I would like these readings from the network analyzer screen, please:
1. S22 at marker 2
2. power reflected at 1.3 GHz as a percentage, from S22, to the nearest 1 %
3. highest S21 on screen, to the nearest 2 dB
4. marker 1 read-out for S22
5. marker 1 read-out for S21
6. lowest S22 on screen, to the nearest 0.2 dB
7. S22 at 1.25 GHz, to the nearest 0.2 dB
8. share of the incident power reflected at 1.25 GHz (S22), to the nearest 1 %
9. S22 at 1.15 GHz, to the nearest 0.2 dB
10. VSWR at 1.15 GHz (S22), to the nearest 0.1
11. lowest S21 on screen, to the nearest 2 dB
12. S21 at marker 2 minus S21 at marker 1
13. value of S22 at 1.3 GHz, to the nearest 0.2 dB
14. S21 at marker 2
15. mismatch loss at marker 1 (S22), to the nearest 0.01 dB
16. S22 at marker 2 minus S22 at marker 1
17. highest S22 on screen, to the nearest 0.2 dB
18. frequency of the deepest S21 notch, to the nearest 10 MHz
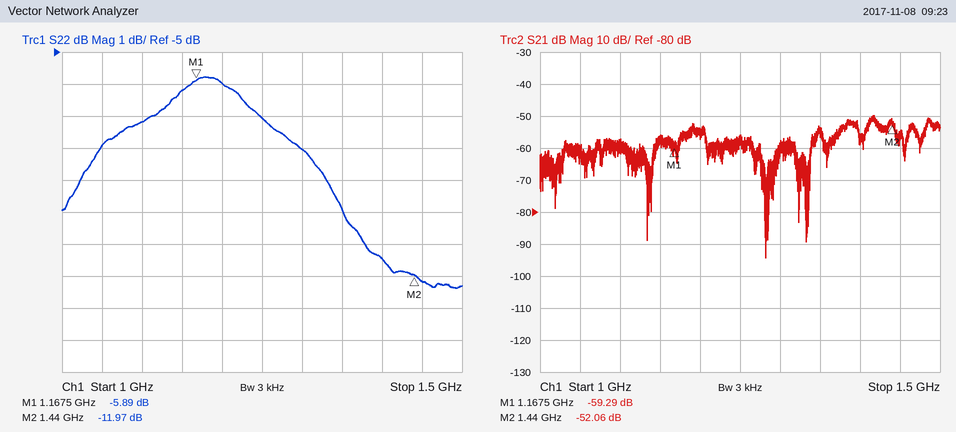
-11.97 dB
16 %
-50 dB
-5.89 dB
-59.29 dB
-12.4 dB
-7.0 dB
20 %
-6.2 dB
2.9
-94 dB
7.23 dB
-8.0 dB
-52.06 dB
1.29 dB
-6.08 dB
-5.8 dB
1.28 GHz
